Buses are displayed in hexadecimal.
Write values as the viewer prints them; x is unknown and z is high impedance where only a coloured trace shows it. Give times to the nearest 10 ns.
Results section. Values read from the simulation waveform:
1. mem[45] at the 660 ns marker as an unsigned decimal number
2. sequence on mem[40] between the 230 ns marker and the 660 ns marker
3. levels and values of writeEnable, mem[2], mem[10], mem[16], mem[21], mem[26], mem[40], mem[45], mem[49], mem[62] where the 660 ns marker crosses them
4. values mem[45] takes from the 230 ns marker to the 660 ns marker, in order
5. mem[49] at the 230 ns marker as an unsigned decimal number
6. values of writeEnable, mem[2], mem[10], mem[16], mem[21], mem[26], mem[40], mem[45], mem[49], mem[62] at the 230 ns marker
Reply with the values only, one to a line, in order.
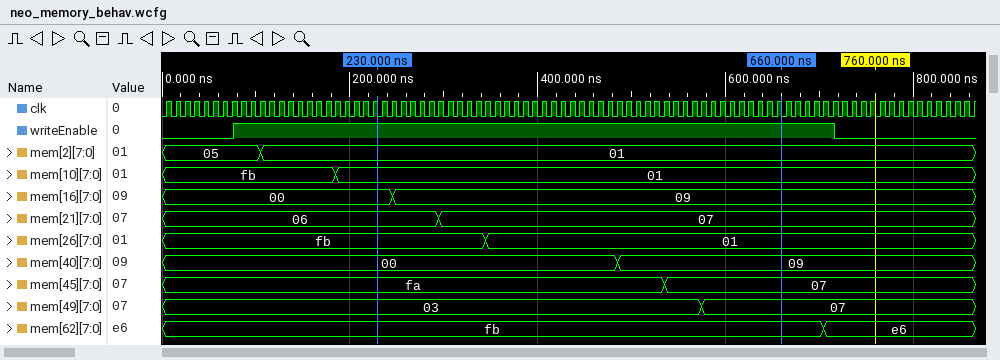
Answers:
7
00, 09
writeEnable=1, mem[2]=01, mem[10]=01, mem[16]=09, mem[21]=07, mem[26]=01, mem[40]=09, mem[45]=07, mem[49]=07, mem[62]=fb
fa, 07
3
writeEnable=1, mem[2]=01, mem[10]=01, mem[16]=00, mem[21]=06, mem[26]=fb, mem[40]=00, mem[45]=fa, mem[49]=03, mem[62]=fb
